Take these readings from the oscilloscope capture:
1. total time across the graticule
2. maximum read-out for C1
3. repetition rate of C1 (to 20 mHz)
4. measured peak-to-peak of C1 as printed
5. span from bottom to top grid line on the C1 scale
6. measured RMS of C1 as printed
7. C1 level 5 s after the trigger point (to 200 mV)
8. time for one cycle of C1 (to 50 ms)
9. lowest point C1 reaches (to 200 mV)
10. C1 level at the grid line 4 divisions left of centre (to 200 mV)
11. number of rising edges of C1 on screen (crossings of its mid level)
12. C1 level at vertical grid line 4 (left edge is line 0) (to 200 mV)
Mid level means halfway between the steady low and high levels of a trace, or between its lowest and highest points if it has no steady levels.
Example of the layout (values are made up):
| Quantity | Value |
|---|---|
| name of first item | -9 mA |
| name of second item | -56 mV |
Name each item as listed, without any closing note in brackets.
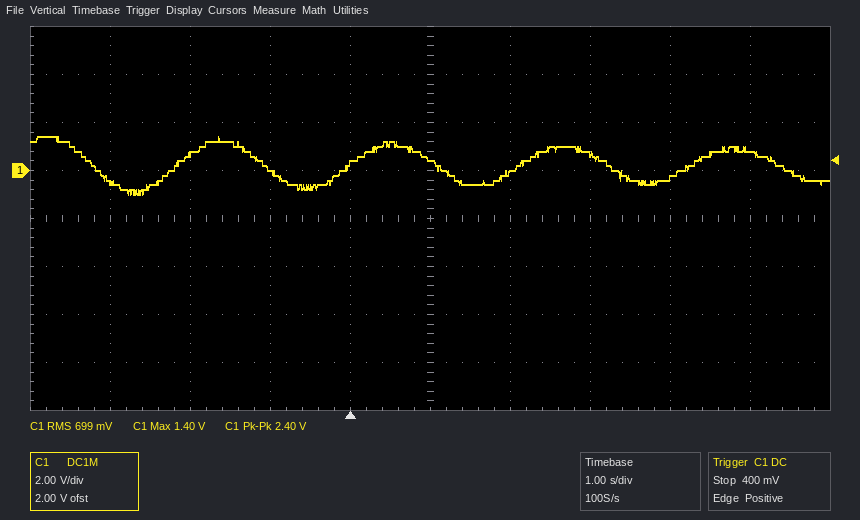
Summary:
| Quantity | Value |
|---|---|
| total time across the graticule | 10 s |
| maximum read-out for C1 | 1.40 V |
| repetition rate of C1 | 460 mHz |
| measured peak-to-peak of C1 as printed | 2.40 V |
| span from bottom to top grid line on the C1 scale | 16 V |
| measured RMS of C1 as printed | 699 mV |
| C1 level 5 s after the trigger point | 800 mV |
| time for one cycle of C1 | 2.15 s |
| lowest point C1 reaches | -1.0 V |
| C1 level at the grid line 4 divisions left of centre | -400 mV |
| number of rising edges of C1 on screen | 4 |
| C1 level at vertical grid line 4 (left edge is line 0) | 200 mV |
